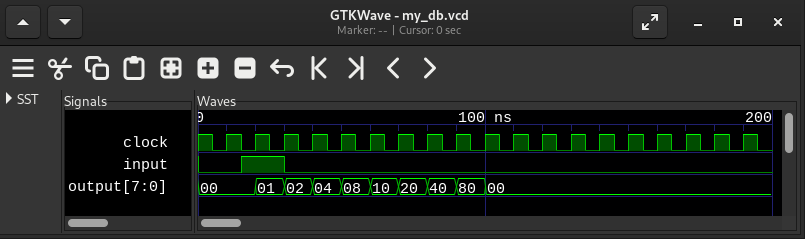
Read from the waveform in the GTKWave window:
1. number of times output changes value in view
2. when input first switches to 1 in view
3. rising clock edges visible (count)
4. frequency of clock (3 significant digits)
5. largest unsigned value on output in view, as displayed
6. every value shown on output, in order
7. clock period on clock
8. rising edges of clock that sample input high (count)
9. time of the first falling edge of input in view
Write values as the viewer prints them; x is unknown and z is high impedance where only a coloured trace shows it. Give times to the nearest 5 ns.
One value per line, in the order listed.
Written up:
9
15 ns
19
100 MHz
80
00, 01, 02, 04, 08, 10, 20, 40, 80, 00
10 ns
2
30 ns
